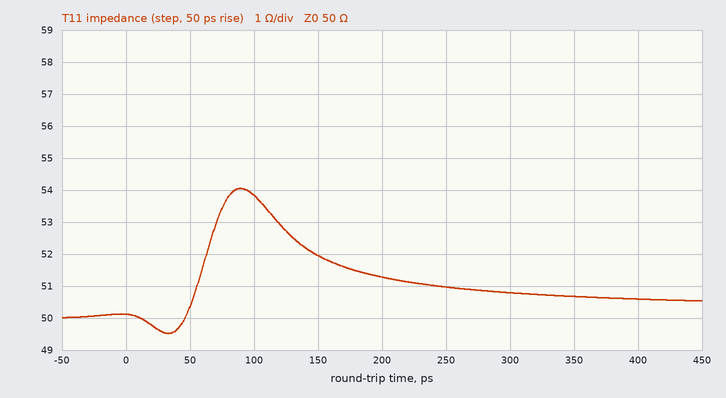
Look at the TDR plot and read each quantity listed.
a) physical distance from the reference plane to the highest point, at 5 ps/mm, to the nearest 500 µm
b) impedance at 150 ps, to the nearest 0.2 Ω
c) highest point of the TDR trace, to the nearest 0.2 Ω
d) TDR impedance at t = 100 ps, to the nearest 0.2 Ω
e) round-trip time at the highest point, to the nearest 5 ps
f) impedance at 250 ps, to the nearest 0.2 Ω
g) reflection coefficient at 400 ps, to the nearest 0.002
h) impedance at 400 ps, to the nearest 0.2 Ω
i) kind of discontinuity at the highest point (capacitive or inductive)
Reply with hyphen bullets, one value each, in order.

- 9.0 mm
- 52.0 Ω
- 54.0 Ω
- 53.8 Ω
- 90 ps
- 51.0 Ω
- +0.006
- 50.6 Ω
- inductive
